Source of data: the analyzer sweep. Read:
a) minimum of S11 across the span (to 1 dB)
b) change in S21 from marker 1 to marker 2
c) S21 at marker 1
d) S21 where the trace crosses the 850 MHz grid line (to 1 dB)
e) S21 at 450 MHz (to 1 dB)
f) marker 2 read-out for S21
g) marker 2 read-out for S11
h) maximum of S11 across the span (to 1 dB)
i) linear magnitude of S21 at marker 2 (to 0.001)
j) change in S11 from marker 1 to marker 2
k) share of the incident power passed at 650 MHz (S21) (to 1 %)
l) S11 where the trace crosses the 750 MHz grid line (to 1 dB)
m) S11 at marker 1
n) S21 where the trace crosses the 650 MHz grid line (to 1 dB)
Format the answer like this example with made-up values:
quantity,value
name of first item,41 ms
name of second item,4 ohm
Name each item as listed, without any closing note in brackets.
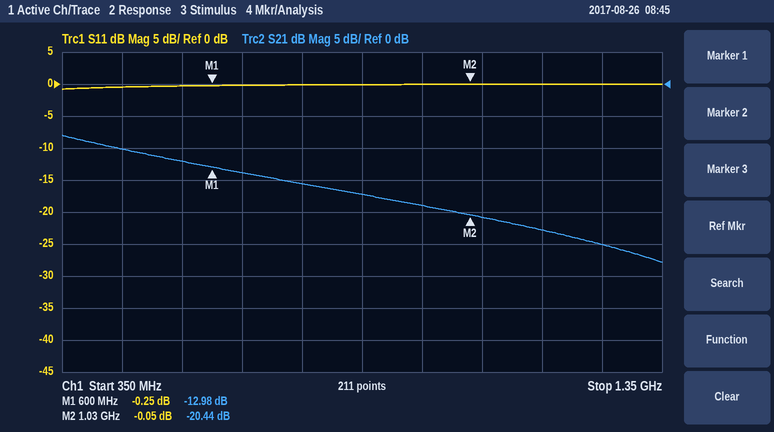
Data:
quantity,value
minimum of S11 across the span,-1 dB
change in S21 from marker 1 to marker 2,-7.46 dB
S21 at marker 1,-12.98 dB
S21 where the trace crosses the 850 MHz grid line,-17 dB
S21 at 450 MHz,-10 dB
marker 2 read-out for S21,-20.44 dB
marker 2 read-out for S11,-0.05 dB
maximum of S11 across the span,0 dB
linear magnitude of S21 at marker 2,0.095
change in S11 from marker 1 to marker 2,0.20 dB
share of the incident power passed at 650 MHz (S21),4 %
S11 where the trace crosses the 750 MHz grid line,0 dB
S11 at marker 1,-0.25 dB
S21 where the trace crosses the 650 MHz grid line,-14 dB
